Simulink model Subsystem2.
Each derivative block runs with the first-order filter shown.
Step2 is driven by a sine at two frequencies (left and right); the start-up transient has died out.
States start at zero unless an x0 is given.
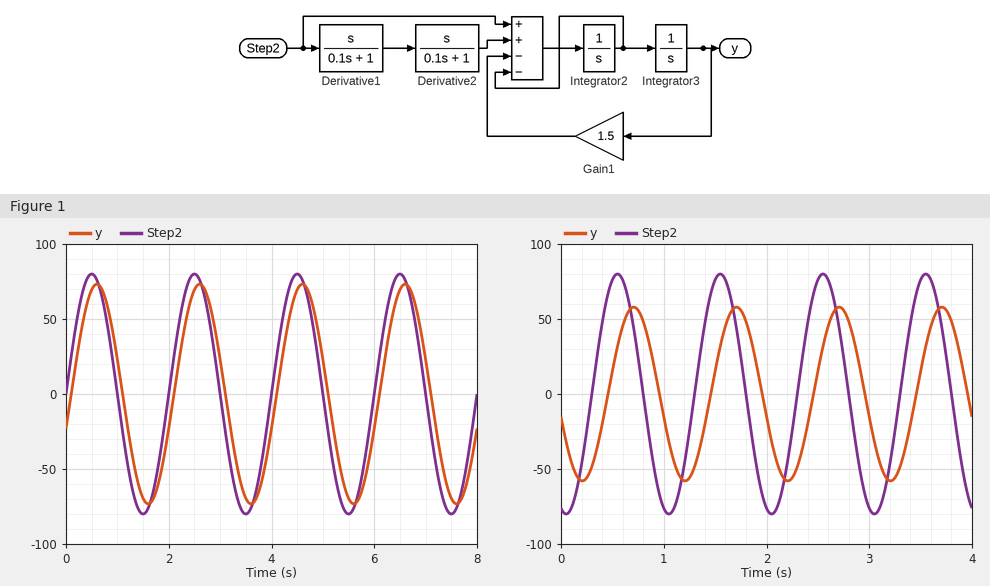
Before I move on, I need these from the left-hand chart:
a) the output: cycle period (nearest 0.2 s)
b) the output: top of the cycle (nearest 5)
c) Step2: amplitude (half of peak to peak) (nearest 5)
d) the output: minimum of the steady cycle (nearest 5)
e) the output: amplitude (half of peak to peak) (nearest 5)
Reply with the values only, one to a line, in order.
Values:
2.0 s
75
80
-75
75
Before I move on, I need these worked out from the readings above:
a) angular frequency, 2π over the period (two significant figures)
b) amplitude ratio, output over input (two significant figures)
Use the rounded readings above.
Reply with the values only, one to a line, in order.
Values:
3.1 rad/s
0.94
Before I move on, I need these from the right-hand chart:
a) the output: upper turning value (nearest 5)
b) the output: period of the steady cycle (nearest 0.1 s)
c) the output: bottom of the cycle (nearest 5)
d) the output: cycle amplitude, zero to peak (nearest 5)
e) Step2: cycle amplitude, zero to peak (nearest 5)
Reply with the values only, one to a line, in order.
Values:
60
1.0 s
-60
60
80
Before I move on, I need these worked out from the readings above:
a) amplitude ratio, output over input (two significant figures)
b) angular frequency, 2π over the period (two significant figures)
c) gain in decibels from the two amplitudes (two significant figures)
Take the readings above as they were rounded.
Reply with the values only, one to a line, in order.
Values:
0.75
6.3 rad/s
-2.5 dB
